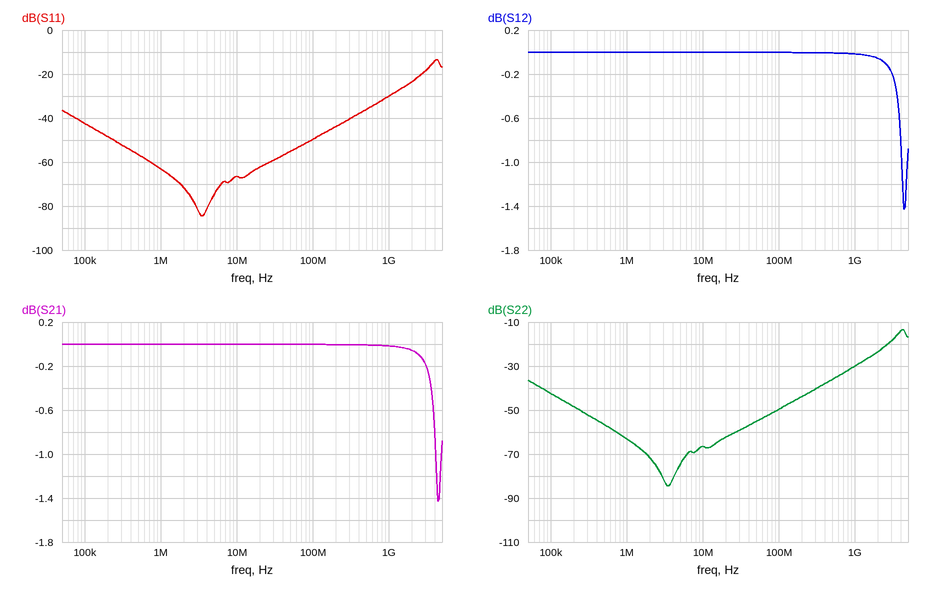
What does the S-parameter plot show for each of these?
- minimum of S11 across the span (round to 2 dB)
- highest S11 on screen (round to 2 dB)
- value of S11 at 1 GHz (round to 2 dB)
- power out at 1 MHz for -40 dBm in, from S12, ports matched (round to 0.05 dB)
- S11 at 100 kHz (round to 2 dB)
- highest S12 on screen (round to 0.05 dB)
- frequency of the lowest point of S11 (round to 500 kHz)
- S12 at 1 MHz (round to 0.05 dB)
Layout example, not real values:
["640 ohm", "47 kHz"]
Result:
["-84 dB", "-14 dB", "-30 dB", "-40.00 dBm", "-42 dB", "0.00 dB", "3.5 MHz", "0.00 dB"]
